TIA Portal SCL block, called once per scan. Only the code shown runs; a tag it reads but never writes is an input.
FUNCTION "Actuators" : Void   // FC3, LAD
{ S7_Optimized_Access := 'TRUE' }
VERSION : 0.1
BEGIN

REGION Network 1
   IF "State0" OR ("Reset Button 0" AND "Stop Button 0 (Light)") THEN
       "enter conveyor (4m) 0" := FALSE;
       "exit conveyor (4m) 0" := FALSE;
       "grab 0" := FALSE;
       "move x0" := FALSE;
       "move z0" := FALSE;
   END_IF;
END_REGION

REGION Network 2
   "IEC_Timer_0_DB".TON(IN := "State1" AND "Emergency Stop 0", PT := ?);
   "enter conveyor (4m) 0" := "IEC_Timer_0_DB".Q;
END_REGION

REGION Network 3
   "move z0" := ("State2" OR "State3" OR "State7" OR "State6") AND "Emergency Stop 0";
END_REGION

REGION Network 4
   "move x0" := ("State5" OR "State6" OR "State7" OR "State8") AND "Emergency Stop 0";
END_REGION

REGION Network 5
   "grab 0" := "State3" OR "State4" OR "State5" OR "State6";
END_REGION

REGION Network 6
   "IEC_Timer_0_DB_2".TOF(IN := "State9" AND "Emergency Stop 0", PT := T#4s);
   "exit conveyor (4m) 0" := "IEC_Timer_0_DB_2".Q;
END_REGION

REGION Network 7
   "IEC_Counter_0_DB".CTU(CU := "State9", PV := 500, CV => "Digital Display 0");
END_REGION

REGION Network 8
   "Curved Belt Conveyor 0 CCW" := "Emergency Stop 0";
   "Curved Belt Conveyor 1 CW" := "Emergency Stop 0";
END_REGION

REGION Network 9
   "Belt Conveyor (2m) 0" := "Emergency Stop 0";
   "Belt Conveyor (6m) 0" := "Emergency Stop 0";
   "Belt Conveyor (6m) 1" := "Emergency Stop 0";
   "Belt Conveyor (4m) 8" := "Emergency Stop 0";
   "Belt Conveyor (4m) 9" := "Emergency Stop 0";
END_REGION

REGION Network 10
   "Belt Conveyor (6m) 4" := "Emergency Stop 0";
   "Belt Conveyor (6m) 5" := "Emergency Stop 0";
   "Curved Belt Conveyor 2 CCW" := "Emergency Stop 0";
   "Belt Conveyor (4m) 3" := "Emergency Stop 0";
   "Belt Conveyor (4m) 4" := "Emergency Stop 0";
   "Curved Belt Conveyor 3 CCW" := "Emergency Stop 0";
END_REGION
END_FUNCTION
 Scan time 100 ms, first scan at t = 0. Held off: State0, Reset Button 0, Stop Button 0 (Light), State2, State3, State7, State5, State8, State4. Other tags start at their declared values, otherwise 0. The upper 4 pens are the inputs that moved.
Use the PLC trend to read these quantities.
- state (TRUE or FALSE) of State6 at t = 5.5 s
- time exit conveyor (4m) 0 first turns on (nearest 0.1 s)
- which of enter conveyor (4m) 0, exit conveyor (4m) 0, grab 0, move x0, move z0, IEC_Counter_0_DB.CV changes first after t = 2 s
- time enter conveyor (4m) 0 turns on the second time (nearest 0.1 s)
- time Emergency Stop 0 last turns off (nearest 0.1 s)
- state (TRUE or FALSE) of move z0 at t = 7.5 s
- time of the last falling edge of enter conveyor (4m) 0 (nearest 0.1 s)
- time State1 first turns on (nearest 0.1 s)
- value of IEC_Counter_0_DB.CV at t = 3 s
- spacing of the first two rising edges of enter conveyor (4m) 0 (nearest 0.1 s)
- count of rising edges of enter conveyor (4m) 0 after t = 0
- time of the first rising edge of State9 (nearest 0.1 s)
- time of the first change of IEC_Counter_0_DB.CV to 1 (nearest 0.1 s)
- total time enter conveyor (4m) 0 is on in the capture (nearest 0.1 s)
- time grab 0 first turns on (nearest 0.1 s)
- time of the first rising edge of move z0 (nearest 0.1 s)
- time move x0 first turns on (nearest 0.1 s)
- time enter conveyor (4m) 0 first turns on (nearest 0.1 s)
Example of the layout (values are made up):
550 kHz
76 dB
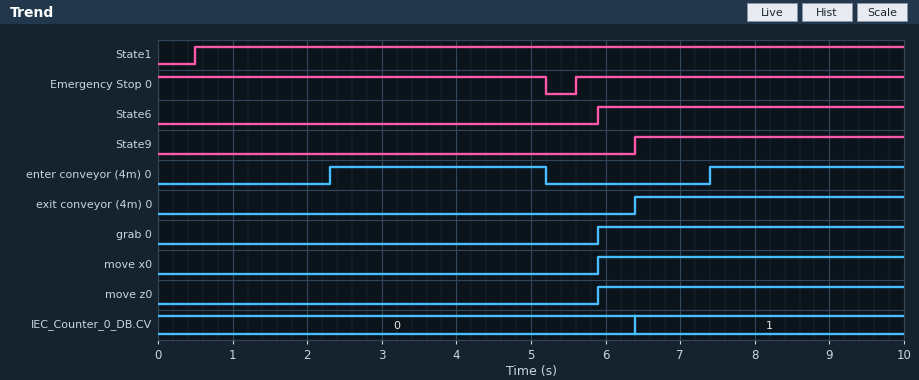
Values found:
FALSE
6.4 s
enter conveyor (4m) 0
7.4 s
5.2 s
TRUE
5.2 s
0.5 s
0
5.1 s
2
6.4 s
6.4 s
5.5 s
5.9 s
5.9 s
5.9 s
2.3 s
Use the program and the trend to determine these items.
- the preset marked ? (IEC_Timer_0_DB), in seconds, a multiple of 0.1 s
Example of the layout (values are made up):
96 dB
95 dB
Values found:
1.8 s
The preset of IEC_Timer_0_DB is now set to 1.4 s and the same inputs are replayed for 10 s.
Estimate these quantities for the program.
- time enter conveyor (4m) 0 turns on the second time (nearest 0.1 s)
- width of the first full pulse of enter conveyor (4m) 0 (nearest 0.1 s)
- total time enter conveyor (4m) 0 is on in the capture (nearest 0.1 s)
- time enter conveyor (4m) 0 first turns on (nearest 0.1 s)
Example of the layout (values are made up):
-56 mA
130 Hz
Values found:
7.0 s
3.3 s
6.3 s
1.9 s
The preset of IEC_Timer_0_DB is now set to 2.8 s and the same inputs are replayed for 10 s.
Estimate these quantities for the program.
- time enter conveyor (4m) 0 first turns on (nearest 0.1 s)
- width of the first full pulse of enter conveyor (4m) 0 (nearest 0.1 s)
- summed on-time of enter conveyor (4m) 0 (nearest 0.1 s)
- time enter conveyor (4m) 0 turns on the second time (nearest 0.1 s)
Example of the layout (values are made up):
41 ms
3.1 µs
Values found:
3.3 s
1.9 s
3.5 s
8.4 s
